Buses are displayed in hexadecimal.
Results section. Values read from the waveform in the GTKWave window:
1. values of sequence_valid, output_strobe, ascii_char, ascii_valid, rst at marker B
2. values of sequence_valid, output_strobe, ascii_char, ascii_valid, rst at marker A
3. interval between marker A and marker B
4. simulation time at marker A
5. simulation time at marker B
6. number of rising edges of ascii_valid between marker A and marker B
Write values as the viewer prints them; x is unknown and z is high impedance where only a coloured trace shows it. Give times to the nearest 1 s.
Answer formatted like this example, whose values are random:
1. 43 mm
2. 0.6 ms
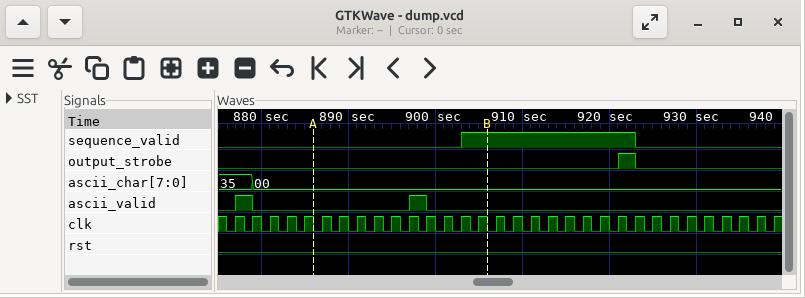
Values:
1. sequence_valid=1, output_strobe=0, ascii_char=00, ascii_valid=0, rst=0
2. sequence_valid=0, output_strobe=0, ascii_char=00, ascii_valid=0, rst=0
3. 20 s
4. 886 s
5. 906 s
6. 1
